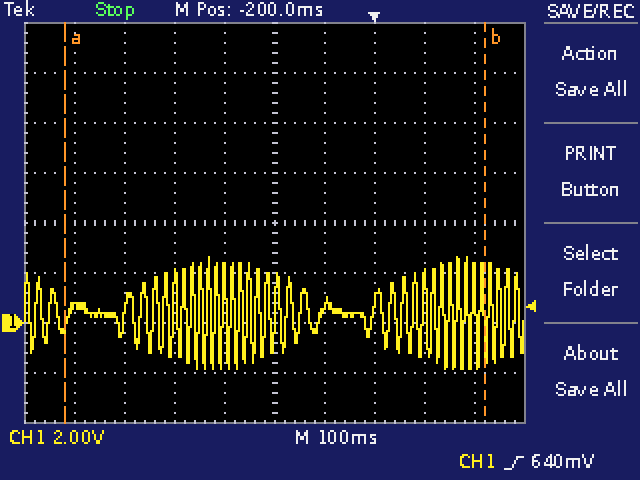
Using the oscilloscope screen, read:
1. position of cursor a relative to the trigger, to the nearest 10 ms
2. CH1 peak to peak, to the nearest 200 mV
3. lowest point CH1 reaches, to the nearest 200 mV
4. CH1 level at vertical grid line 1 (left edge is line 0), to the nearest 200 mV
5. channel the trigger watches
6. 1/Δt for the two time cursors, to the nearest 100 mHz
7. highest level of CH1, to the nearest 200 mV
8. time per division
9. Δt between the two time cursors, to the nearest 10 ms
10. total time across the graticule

-620 ms
4.4 V
-1.8 V
600 mV
CH1
1.2 Hz
2.6 V
100 ms
840 ms
1 s
